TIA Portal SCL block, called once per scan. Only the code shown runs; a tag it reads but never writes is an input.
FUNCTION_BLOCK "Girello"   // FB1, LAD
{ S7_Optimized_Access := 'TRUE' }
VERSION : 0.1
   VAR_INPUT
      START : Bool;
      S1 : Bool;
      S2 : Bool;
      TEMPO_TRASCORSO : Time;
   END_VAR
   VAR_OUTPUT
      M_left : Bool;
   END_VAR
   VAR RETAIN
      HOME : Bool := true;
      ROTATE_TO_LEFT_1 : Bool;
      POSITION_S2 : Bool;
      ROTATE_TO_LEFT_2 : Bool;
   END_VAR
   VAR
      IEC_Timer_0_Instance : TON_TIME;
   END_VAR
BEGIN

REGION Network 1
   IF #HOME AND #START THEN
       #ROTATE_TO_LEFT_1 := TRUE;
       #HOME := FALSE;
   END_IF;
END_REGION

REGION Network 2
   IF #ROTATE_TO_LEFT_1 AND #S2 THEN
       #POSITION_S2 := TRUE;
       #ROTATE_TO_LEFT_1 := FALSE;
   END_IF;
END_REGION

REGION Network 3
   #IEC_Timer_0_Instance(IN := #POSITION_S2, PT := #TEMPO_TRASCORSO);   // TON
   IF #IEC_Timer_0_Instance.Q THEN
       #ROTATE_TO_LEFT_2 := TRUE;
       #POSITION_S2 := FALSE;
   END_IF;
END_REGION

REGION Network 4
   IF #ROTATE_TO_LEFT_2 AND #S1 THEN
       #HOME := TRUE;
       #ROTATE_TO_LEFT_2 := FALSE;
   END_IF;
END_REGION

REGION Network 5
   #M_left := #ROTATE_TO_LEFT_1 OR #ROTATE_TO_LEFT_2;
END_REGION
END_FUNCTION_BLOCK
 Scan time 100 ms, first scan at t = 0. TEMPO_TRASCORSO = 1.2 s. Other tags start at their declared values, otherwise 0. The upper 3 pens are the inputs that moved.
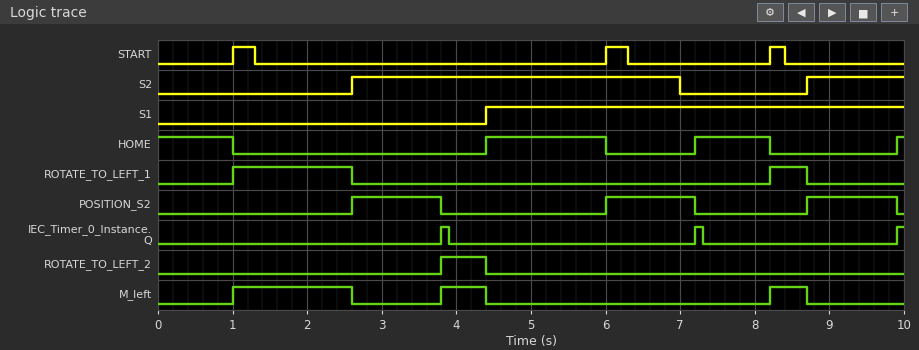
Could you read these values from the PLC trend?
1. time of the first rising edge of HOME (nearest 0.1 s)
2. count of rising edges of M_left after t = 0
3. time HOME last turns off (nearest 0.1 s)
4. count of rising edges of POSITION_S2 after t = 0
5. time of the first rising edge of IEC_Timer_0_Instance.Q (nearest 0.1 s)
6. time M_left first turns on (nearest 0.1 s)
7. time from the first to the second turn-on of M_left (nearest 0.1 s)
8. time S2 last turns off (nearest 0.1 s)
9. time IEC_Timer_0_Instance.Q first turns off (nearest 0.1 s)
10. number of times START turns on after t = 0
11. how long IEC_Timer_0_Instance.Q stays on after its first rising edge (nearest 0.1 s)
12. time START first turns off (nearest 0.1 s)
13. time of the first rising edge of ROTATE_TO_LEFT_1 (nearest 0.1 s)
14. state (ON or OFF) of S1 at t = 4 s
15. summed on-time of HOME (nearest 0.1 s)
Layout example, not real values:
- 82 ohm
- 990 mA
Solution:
- 4.4 s
- 3
- 8.2 s
- 3
- 3.8 s
- 1.0 s
- 2.8 s
- 7.0 s
- 3.9 s
- 3
- 0.1 s
- 1.3 s
- 1.0 s
- OFF
- 3.7 s
